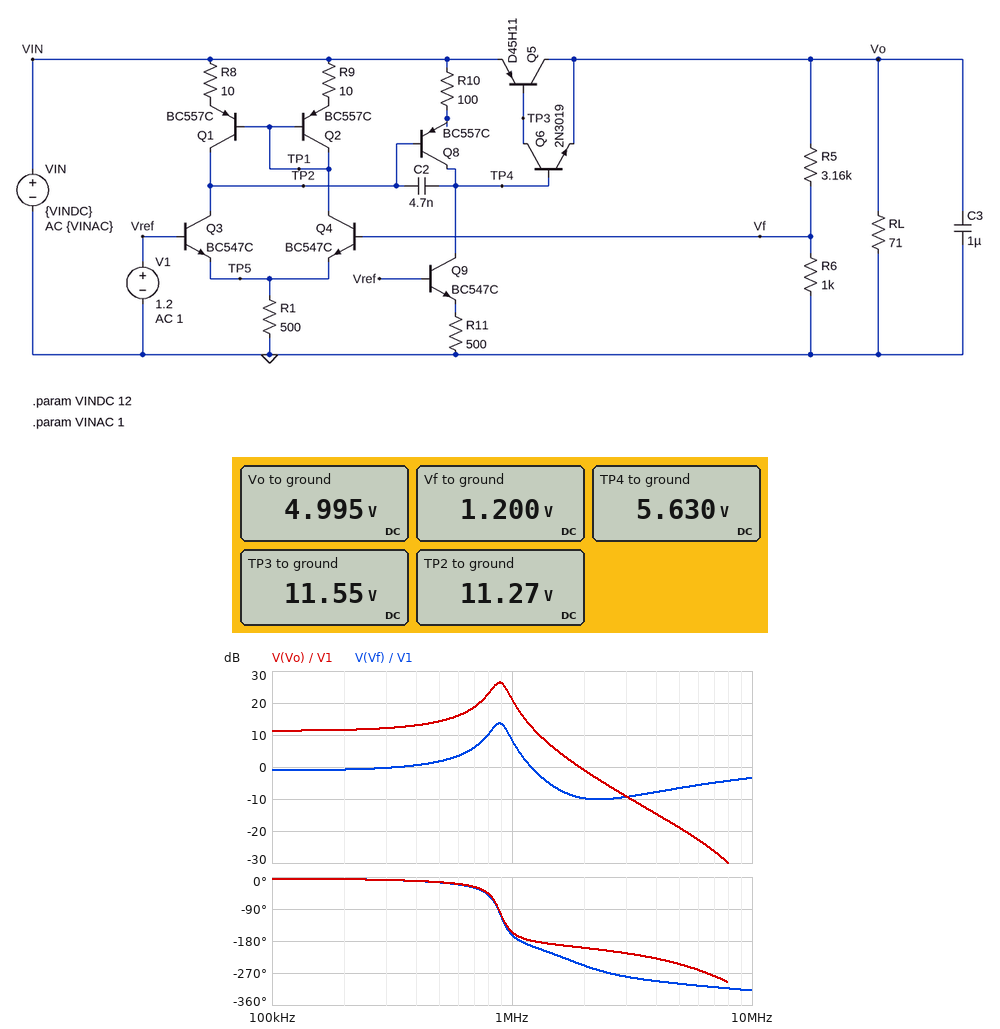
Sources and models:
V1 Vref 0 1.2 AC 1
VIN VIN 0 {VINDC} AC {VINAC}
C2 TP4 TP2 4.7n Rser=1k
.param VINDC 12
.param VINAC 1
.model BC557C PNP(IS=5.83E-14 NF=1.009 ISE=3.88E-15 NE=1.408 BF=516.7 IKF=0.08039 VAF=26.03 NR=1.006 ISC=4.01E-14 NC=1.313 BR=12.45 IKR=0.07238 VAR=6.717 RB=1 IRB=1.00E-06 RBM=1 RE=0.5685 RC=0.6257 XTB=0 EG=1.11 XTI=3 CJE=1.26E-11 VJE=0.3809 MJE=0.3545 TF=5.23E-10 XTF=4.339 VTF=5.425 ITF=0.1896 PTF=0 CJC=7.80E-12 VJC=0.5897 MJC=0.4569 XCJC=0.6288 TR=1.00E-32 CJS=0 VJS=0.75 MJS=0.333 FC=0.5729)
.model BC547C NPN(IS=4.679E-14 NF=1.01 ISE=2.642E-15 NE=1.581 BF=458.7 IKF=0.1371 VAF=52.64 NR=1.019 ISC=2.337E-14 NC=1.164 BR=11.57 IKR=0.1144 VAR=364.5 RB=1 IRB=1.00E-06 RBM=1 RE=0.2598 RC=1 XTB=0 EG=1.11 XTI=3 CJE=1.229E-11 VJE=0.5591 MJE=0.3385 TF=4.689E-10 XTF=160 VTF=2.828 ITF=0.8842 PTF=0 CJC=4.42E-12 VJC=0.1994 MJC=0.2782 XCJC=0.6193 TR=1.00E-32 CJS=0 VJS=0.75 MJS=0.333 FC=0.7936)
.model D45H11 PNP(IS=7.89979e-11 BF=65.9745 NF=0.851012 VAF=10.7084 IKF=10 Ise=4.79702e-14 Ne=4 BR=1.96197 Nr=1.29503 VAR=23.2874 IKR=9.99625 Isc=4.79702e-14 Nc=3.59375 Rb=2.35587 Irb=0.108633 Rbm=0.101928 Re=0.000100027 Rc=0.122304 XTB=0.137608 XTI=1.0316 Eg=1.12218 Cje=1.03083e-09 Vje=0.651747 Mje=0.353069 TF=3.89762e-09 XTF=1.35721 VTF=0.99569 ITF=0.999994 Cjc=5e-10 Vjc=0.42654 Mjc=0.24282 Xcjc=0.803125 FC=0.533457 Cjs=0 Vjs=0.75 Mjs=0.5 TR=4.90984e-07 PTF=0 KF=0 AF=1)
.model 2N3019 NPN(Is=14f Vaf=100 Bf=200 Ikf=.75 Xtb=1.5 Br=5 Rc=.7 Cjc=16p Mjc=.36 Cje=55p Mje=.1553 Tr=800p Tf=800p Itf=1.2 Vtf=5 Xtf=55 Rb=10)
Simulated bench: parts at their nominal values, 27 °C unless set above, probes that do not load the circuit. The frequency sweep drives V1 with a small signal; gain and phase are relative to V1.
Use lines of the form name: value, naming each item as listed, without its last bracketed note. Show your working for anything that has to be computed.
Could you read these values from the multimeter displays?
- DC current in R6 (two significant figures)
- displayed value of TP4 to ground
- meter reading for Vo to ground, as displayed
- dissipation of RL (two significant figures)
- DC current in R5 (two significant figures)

DC current in R6: (1.2 V) / 1 kΩ = 1.2 mA
displayed value of TP4 to ground: 5.630 V
meter reading for Vo to ground, as displayed: 4.995 V
dissipation of RL: (4.995 V)^2 / 71 Ω = 350 mW
DC current in R5: (4.995 V - 1.2 V) / 3.16 kΩ = 1.2 mA
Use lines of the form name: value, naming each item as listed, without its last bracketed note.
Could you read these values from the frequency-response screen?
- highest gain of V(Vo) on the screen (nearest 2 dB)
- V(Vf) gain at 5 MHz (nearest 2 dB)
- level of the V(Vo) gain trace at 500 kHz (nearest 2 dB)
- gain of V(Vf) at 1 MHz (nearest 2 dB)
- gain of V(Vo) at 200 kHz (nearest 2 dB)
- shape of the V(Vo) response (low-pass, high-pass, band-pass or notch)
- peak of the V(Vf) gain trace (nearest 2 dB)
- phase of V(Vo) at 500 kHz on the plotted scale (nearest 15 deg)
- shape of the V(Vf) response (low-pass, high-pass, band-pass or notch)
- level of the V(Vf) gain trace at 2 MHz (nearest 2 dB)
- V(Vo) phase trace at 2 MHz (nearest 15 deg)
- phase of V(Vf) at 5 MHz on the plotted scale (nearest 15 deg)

highest gain of V(Vo) on the screen: 26 dB
V(Vf) gain at 5 MHz: -6 dB
level of the V(Vo) gain trace at 500 kHz: 14 dB
gain of V(Vf) at 1 MHz: 8 dB
gain of V(Vo) at 200 kHz: 12 dB
shape of the V(Vo) response: low-pass
peak of the V(Vf) gain trace: 14 dB
phase of V(Vo) at 500 kHz on the plotted scale: -15 deg
shape of the V(Vf) response: band-pass
level of the V(Vf) gain trace at 2 MHz: -10 dB
V(Vo) phase trace at 2 MHz: -195 deg
phase of V(Vf) at 5 MHz on the plotted scale: -300 deg
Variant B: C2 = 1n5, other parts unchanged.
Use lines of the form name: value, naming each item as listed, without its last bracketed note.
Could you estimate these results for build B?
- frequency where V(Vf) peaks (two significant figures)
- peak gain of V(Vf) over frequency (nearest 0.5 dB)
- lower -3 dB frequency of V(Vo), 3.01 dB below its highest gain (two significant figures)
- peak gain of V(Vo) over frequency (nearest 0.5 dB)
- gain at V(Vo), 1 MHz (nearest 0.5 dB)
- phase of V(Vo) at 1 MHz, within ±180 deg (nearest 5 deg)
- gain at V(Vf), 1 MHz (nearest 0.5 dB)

frequency where V(Vf) peaks: 880 kHz
peak gain of V(Vf) over frequency: 19.0 dB
lower -3 dB frequency of V(Vo), 3.01 dB below its highest gain: 840 kHz
peak gain of V(Vo) over frequency: 31.5 dB
gain at V(Vo), 1 MHz: 22.0 dB
phase of V(Vo) at 1 MHz, within ±180 deg: -170 deg
gain at V(Vf), 1 MHz: 9.0 dB
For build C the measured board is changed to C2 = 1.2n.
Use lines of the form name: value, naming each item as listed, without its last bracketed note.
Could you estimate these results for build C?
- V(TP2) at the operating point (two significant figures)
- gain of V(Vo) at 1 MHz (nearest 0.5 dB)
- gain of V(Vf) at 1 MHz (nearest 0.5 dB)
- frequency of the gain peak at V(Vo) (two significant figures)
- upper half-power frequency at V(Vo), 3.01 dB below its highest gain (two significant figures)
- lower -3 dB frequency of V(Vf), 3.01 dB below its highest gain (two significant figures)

V(TP2) at the operating point: 11 V
gain of V(Vo) at 1 MHz: 22.0 dB
gain of V(Vf) at 1 MHz: 9.5 dB
frequency of the gain peak at V(Vo): 880 kHz
upper half-power frequency at V(Vo), 3.01 dB below its highest gain: 910 kHz
lower -3 dB frequency of V(Vf), 3.01 dB below its highest gain: 850 kHz
